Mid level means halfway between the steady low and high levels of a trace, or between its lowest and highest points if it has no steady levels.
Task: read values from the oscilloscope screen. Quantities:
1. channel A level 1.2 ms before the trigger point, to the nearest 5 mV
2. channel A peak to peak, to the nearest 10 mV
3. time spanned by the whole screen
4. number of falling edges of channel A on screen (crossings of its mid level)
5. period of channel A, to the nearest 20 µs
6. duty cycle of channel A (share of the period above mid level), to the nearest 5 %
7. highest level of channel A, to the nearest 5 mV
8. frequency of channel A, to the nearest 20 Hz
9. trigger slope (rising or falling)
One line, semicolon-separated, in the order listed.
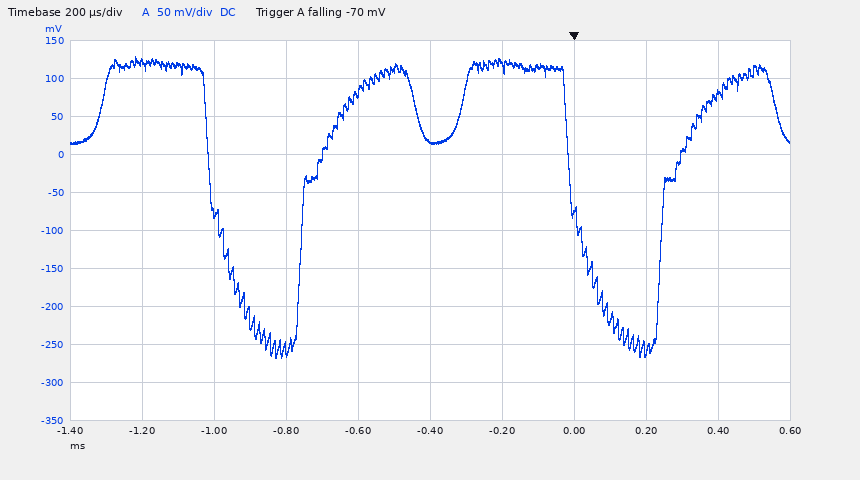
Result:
120 mV; 400 mV; 2 ms; 2; 1.00 ms; 75 %; 130 mV; 1.00 kHz; falling
